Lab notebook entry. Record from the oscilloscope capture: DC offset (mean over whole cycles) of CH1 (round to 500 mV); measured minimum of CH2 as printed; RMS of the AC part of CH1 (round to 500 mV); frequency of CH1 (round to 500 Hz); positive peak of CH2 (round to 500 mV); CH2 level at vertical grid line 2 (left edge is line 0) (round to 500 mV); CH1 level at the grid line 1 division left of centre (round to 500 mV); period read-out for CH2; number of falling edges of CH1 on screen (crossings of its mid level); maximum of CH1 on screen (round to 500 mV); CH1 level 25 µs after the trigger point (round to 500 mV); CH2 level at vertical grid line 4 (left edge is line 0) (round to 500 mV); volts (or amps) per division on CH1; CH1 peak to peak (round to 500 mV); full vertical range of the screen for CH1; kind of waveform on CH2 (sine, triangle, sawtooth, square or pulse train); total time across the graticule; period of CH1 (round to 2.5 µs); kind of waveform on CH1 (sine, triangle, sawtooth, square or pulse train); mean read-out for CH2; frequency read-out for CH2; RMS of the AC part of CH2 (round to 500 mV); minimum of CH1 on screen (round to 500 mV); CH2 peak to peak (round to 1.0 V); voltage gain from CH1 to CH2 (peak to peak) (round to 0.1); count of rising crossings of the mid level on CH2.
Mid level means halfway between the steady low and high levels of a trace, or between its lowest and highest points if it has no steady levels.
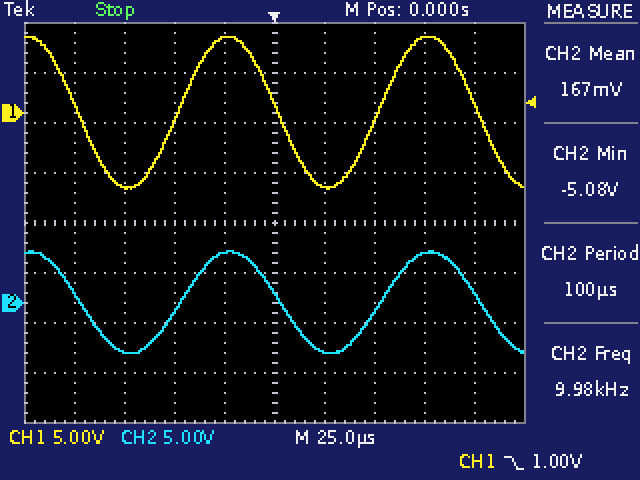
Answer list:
0.0 V
-5.08 V
5.5 V
10.0 kHz
5.0 V
-5.0 V
7.5 V
100 µs
3
7.5 V
-7.5 V
5.0 V
5 V
15.0 V
40 V
sine
250 µs
100.0 µs
sine
167 mV
9.98 kHz
3.5 V
-7.5 V
10.0 V
0.7
2
